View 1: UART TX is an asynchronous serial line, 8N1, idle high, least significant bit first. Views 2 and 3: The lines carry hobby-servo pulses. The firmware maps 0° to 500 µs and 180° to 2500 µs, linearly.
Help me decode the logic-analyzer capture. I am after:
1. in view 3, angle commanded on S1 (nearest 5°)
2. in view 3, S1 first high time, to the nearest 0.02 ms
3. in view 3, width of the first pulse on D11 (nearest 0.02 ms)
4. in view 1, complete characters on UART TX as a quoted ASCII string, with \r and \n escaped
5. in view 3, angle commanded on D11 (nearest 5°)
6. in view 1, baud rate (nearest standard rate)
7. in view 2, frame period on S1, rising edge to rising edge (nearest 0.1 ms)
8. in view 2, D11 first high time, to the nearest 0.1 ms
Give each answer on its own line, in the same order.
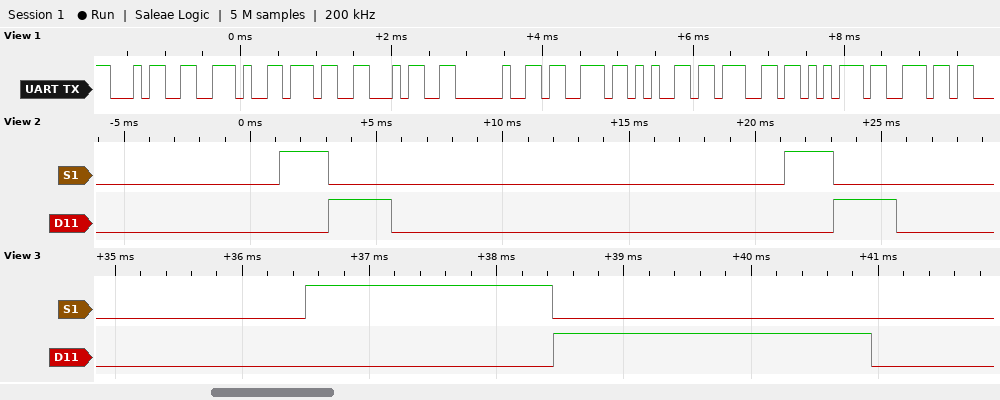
130°
1.94 ms
2.50 ms
"4.74 segun"
180°
9600 baud
20.0 ms
2.5 ms
